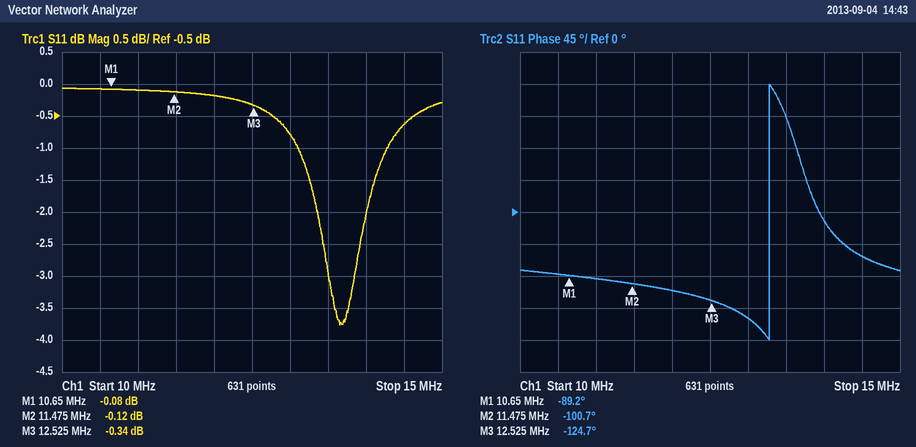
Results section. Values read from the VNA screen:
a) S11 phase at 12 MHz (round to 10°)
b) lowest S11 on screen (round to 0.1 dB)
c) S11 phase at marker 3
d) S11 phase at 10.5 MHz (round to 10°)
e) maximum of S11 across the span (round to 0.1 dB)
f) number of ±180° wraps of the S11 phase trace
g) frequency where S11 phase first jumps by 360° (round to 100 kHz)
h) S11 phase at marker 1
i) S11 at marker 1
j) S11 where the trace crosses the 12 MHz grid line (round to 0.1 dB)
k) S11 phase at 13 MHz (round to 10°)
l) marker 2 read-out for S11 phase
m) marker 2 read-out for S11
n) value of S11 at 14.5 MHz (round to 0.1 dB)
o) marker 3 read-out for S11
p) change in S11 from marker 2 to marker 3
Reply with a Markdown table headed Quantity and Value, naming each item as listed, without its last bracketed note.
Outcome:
| Quantity | Value |
|---|---|
| S11 phase at 12 MHz | -110° |
| lowest S11 on screen | -3.8 dB |
| S11 phase at marker 3 | -124.7° |
| S11 phase at 10.5 MHz | -90° |
| maximum of S11 across the span | -0.1 dB |
| number of ±180° wraps of the S11 phase trace | 1 |
| frequency where S11 phase first jumps by 360° | 13.3 MHz |
| S11 phase at marker 1 | -89.2° |
| S11 at marker 1 | -0.08 dB |
| S11 where the trace crosses the 12 MHz grid line | -0.2 dB |
| S11 phase at 13 MHz | -150° |
| marker 2 read-out for S11 phase | -100.7° |
| marker 2 read-out for S11 | -0.12 dB |
| value of S11 at 14.5 MHz | -0.6 dB |
| marker 3 read-out for S11 | -0.34 dB |
| change in S11 from marker 2 to marker 3 | -0.22 dB |
